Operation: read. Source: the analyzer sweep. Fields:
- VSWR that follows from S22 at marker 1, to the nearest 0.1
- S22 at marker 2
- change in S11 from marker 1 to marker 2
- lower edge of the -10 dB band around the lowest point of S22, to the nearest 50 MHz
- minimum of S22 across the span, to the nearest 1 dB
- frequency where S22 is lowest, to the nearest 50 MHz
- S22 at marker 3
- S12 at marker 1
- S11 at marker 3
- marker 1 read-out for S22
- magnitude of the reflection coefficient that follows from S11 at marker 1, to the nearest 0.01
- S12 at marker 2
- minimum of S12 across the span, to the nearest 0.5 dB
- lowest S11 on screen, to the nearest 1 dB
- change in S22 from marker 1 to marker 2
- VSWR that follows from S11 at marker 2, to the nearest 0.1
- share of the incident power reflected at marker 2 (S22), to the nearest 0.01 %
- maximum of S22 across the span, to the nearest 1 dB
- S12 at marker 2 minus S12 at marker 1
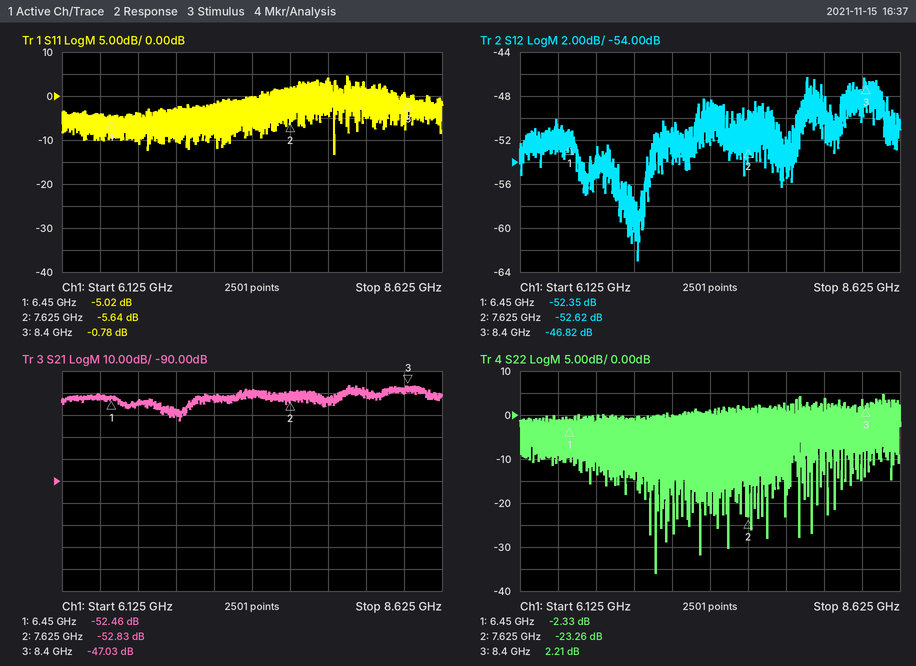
7.5
-23.26 dB
-0.62 dB
7.00 GHz
-36 dB
7.00 GHz
2.21 dB
-52.35 dB
-0.78 dB
-2.33 dB
0.56
-52.62 dB
-63.0 dB
-13 dB
-20.93 dB
3.2
0.47 %
5 dB
-0.27 dB
